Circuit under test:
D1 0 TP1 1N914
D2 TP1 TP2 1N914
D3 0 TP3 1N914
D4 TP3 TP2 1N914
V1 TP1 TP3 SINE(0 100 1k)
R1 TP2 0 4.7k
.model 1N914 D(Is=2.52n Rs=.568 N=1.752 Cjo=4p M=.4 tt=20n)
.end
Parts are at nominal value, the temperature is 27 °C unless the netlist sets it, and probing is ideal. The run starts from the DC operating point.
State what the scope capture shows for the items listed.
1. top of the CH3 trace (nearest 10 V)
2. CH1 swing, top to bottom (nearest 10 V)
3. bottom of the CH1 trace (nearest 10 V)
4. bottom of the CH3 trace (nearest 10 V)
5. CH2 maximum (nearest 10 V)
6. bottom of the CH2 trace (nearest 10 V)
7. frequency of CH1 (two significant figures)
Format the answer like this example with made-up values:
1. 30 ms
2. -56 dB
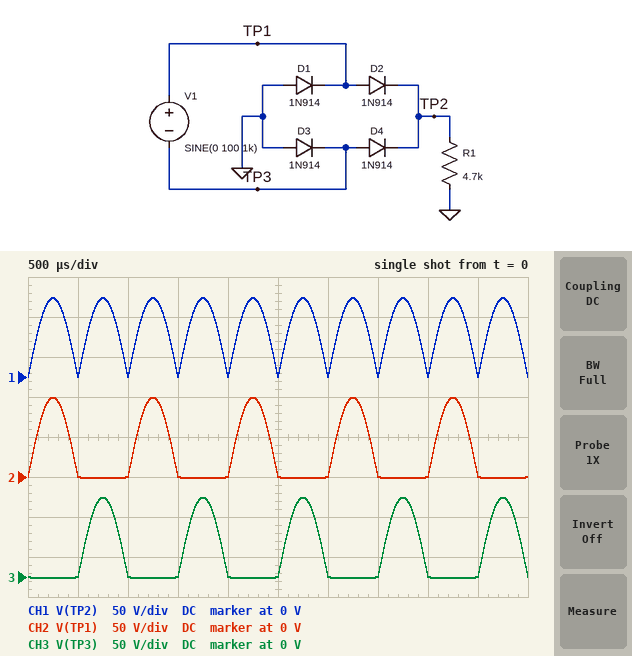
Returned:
1. 100 V
2. 100 V
3. 0 V
4. 0 V
5. 100 V
6. 0 V
7. 2.0 kHz
